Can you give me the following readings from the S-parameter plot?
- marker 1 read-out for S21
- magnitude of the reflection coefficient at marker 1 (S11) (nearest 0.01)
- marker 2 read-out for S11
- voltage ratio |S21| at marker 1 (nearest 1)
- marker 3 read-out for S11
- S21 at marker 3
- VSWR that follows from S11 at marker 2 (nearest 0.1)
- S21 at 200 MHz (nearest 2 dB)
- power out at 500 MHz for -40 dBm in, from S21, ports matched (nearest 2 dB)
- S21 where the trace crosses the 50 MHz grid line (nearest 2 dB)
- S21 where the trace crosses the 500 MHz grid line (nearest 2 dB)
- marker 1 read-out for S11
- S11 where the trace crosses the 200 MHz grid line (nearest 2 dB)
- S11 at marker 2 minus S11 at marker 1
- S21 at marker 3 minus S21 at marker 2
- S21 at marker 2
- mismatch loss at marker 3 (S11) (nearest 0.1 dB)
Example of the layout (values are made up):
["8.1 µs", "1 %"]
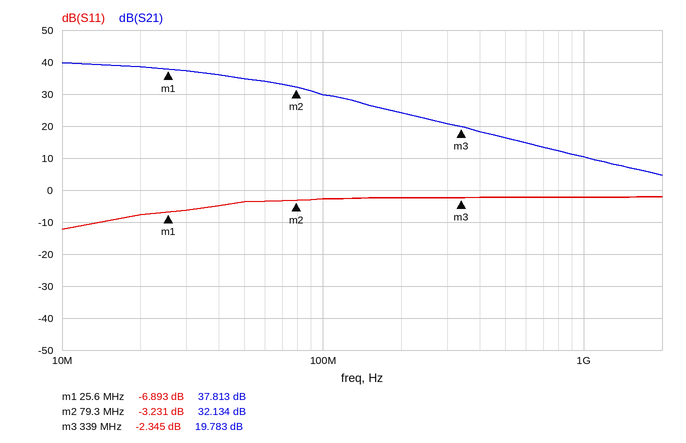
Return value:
["37.813 dB", "0.45", "-3.231 dB", "78", "-2.345 dB", "19.783 dB", "5.4", "24 dB", "-24 dBm", "34 dB", "16 dB", "-6.893 dB", "-2 dB", "3.662 dB", "-12.351 dB", "32.134 dB", "3.8 dB"]
